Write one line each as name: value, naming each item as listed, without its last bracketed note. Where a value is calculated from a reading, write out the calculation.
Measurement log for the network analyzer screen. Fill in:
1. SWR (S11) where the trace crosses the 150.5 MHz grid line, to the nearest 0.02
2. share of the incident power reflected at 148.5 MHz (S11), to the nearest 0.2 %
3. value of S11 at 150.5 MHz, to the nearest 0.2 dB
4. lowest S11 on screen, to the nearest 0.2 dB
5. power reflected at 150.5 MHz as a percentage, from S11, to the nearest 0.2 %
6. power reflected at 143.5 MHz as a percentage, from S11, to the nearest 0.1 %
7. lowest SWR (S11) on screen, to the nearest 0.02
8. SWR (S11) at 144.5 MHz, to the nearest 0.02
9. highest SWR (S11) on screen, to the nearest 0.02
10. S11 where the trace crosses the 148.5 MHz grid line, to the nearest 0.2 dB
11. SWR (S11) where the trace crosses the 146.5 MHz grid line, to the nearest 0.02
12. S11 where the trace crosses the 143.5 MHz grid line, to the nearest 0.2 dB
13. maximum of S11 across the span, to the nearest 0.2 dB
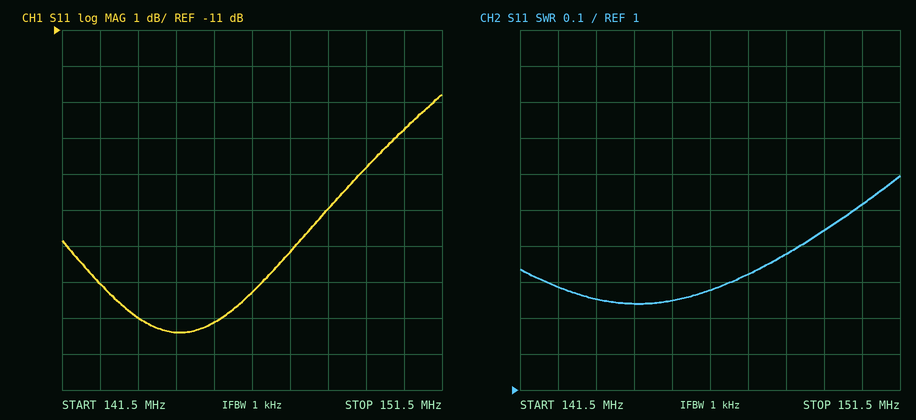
SWR (S11) where the trace crosses the 150.5 MHz grid line, to the nearest 0.02: 1.52
share of the incident power reflected at 148.5 MHz (S11), to the nearest 0.2 %: 10^(-16/10) ≈ 2.51 %, so 2.6 % to the nearest 0.2 %
value of S11 at 150.5 MHz, to the nearest 0.2 dB: -13.8 dB
lowest S11 on screen, to the nearest 0.2 dB: -19.4 dB
power reflected at 150.5 MHz as a percentage, from S11, to the nearest 0.2 %: 10^(-13.8/10) ≈ 4.2 %
power reflected at 143.5 MHz as a percentage, from S11, to the nearest 0.1 %: 10^(-19/10) ≈ 1.3 %
lowest SWR (S11) on screen, to the nearest 0.02: 1.24
SWR (S11) at 144.5 MHz, to the nearest 0.02: 1.24
highest SWR (S11) on screen, to the nearest 0.02: 1.60
S11 where the trace crosses the 148.5 MHz grid line, to the nearest 0.2 dB: -16.0 dB
SWR (S11) where the trace crosses the 146.5 MHz grid line, to the nearest 0.02: 1.28
S11 where the trace crosses the 143.5 MHz grid line, to the nearest 0.2 dB: -19.0 dB
maximum of S11 across the span, to the nearest 0.2 dB: -12.8 dB
